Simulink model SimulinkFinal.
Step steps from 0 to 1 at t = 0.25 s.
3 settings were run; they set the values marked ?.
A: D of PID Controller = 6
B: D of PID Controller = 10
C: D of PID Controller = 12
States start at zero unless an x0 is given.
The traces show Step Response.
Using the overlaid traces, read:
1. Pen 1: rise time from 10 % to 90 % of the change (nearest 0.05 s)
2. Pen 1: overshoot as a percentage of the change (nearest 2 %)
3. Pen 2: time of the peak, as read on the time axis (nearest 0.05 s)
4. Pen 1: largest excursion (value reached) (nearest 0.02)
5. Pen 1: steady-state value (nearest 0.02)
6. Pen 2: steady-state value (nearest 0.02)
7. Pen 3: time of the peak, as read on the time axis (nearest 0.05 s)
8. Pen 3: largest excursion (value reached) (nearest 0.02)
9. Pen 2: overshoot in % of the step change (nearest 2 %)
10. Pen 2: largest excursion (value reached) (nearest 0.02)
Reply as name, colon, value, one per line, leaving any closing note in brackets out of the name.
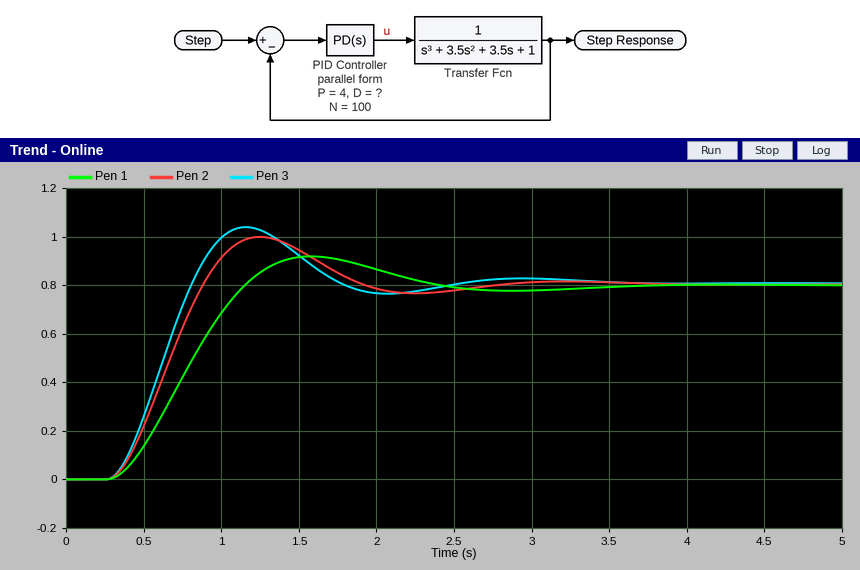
Pen 1: rise time from 10 % to 90 % of the change: 0.60 s
Pen 1: overshoot as a percentage of the change: 14 %
Pen 2: time of the peak, as read on the time axis: 1.25 s
Pen 1: largest excursion (value reached): 0.92
Pen 1: steady-state value: 0.80
Pen 2: steady-state value: 0.80
Pen 3: time of the peak, as read on the time axis: 1.15 s
Pen 3: largest excursion (value reached): 1.04
Pen 2: overshoot in % of the step change: 24 %
Pen 2: largest excursion (value reached): 1.00
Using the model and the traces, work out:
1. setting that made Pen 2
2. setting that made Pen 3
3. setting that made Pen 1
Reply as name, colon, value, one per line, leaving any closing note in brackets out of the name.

setting that made Pen 2: B
setting that made Pen 3: C
setting that made Pen 1: A
